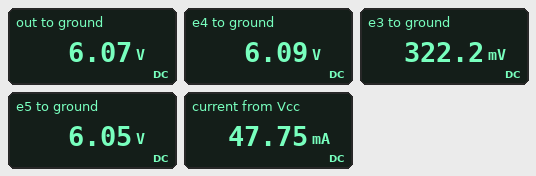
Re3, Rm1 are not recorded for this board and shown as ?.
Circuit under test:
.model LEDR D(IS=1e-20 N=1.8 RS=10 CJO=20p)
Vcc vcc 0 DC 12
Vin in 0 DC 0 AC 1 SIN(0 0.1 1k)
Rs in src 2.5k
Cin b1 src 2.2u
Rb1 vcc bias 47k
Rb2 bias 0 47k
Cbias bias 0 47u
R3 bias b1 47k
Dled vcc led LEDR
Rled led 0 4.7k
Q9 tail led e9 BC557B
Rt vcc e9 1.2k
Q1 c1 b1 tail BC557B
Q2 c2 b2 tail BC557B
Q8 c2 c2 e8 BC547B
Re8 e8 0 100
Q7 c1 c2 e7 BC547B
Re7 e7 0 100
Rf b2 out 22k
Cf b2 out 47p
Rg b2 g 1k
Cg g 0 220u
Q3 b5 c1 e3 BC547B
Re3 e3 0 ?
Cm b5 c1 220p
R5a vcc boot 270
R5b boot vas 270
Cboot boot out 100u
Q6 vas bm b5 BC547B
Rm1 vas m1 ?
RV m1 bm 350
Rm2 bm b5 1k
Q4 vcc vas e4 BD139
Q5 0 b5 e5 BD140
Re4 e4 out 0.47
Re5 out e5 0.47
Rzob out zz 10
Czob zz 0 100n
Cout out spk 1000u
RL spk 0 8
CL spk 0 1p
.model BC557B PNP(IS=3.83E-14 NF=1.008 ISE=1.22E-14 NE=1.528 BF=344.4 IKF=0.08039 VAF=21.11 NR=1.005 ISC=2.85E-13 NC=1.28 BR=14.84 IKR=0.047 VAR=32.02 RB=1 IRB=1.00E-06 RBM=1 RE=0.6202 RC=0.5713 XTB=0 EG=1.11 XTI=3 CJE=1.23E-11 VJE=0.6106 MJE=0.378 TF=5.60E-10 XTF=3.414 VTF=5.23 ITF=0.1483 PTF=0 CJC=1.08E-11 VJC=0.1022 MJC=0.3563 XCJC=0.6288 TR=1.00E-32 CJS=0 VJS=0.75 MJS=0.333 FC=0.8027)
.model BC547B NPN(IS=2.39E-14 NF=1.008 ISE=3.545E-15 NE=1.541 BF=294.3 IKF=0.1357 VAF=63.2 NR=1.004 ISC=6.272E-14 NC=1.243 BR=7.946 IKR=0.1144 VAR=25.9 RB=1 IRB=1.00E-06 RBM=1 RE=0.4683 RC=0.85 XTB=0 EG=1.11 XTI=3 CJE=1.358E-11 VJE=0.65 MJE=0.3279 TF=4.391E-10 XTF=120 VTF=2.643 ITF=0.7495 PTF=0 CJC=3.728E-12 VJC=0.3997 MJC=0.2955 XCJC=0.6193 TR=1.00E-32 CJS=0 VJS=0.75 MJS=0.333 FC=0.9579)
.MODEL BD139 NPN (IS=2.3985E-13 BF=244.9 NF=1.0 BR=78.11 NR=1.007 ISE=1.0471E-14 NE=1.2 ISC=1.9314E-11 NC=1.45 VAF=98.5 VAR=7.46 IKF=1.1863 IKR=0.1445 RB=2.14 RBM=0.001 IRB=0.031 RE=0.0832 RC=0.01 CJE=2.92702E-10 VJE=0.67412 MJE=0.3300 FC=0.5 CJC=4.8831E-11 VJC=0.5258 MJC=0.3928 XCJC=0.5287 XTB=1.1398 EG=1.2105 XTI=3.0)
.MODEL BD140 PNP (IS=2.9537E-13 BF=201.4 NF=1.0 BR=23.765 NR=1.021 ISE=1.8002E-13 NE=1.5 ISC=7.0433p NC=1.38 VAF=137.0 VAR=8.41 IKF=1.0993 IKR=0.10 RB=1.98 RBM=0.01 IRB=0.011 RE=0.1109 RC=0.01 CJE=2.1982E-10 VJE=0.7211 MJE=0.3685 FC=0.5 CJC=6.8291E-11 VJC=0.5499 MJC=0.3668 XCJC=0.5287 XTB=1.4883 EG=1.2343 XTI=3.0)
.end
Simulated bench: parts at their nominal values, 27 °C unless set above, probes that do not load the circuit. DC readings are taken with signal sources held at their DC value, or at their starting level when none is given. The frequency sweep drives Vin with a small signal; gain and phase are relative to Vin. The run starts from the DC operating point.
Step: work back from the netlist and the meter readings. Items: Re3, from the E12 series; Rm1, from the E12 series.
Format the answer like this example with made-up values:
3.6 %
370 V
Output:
33 Ω
560 Ω
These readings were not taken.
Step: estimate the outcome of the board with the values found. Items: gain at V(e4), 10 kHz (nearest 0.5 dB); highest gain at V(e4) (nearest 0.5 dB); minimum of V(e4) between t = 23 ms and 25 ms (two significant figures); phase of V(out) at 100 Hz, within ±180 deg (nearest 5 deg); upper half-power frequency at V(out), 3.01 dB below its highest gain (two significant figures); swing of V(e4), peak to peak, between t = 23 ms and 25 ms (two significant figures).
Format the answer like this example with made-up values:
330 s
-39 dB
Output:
27.0 dB
27.0 dB
3.9 V
0 deg
120 kHz
4.5 V
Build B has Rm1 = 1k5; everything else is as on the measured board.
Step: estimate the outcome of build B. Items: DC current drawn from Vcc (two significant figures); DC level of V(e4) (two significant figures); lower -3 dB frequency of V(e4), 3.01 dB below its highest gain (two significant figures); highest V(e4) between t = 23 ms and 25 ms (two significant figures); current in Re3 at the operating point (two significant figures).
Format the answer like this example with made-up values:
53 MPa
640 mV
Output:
460 mA
6.3 V
2.0 Hz
8.5 V
9.6 mA
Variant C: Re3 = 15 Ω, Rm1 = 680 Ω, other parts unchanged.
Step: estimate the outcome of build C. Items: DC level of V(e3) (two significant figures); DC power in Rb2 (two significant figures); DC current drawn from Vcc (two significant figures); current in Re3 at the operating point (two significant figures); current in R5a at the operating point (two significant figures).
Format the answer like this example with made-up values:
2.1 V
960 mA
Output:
150 mV
770 µW
86 mA
9.7 mA
9.6 mA
